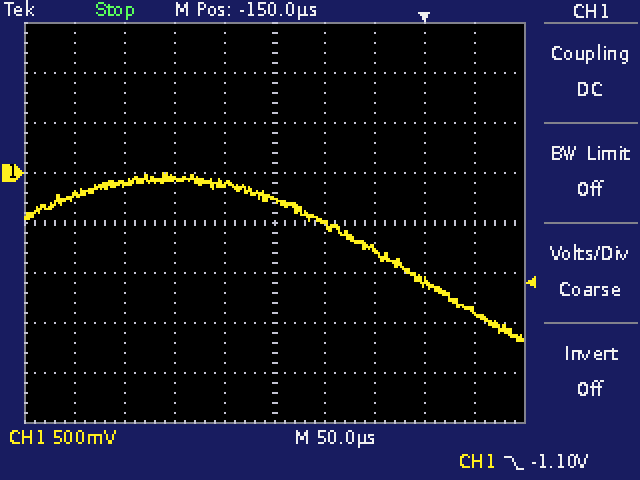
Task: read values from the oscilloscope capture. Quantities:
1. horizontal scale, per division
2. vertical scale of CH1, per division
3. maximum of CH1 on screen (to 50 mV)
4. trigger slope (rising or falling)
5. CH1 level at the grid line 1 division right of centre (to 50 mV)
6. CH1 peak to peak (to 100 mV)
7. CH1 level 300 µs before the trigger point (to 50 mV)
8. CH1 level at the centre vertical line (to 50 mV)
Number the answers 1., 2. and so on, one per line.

1. 50 µs
2. 500 mV
3. 0 mV
4. falling
5. -500 mV
6. 1.70 V
7. -100 mV
8. -250 mV
